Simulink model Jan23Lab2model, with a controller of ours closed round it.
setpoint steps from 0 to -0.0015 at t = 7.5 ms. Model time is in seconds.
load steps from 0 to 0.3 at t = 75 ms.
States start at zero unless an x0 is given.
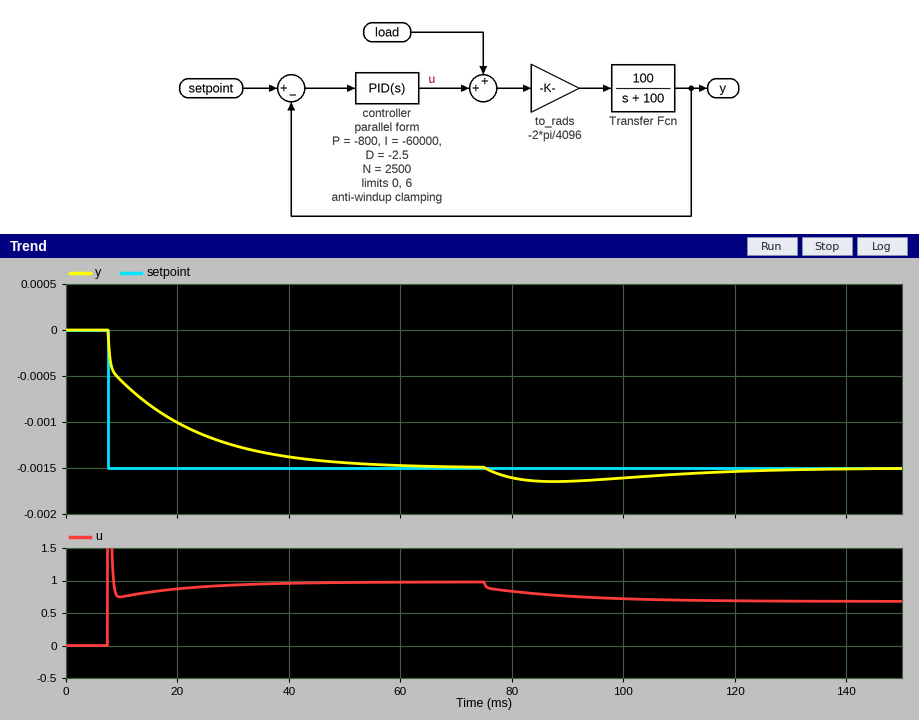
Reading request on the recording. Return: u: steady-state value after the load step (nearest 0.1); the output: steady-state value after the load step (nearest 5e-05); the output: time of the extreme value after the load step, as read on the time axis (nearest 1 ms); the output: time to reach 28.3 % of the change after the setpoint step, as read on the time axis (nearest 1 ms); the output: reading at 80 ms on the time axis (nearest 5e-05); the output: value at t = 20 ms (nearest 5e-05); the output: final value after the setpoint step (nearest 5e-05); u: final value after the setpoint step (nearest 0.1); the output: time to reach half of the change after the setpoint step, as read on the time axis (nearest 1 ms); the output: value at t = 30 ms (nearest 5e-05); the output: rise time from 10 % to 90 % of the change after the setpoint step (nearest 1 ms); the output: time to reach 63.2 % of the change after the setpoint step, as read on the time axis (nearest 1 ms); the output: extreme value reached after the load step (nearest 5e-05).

0.7
-0.00150
88 ms
8 ms
-0.00160
-0.00100
-0.00150
1.0
14 ms
-0.00125
29 ms
18 ms
-0.00165
